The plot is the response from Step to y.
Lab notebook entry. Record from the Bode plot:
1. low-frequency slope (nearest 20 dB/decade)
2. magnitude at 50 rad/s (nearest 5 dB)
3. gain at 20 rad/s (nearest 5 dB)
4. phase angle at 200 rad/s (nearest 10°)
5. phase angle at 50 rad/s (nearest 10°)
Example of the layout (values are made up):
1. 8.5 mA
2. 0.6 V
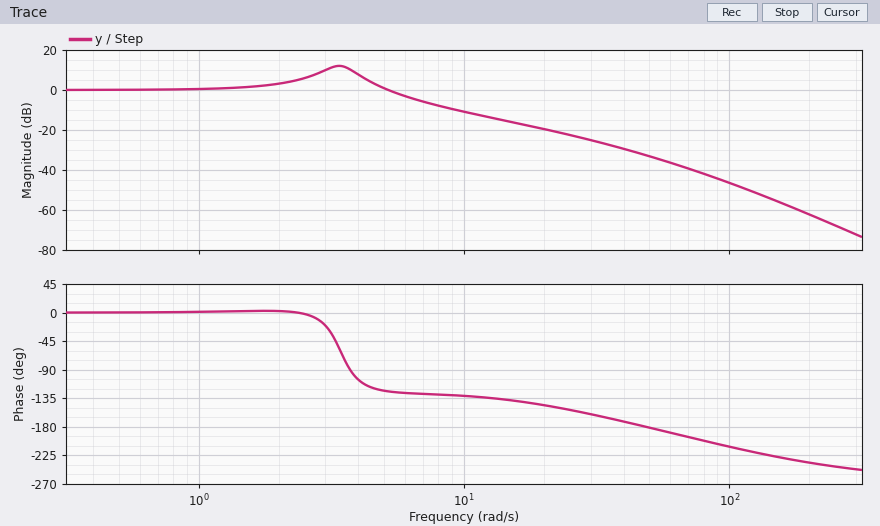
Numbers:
1. 0 dB/decade
2. -35 dB
3. -20 dB
4. -240°
5. -180°
